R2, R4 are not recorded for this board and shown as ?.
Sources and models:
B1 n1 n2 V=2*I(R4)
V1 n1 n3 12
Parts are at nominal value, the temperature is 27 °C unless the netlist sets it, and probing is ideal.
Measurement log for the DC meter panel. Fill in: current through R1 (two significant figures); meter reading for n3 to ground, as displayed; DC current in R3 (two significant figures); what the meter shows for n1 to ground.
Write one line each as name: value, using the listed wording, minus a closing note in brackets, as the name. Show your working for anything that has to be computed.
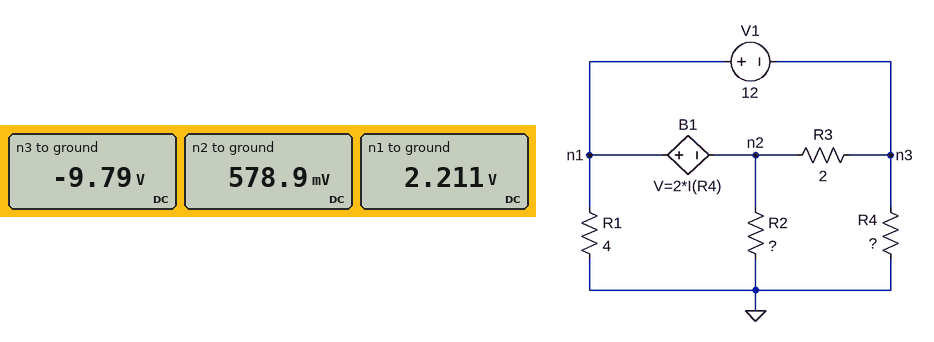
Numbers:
current through R1: (2.211 V) / 4 Ω = 550 mA
meter reading for n3 to ground, as displayed: -9.79 V
DC current in R3: (578.9 mV - (-9.79 V)) / 2 Ω = 5.2 A
what the meter shows for n1 to ground: 2.211 V
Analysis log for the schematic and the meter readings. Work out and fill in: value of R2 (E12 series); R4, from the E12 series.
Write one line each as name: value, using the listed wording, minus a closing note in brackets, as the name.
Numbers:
value of R2: 2.2 Ω
R4, from the E12 series: 12 Ω
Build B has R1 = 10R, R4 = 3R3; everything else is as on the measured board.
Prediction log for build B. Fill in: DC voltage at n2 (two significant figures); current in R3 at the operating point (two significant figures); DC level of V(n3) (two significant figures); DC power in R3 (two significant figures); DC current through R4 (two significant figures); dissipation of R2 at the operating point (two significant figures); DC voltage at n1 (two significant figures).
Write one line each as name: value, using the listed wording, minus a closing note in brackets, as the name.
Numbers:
DC voltage at n2: 2.6 V
current in R3 at the operating point: 4.2 A
DC level of V(n3): -5.9 V
DC power in R3: 36 W
DC current through R4: 1.8 A
dissipation of R2 at the operating point: 3.0 W
DC voltage at n1: 6.1 V
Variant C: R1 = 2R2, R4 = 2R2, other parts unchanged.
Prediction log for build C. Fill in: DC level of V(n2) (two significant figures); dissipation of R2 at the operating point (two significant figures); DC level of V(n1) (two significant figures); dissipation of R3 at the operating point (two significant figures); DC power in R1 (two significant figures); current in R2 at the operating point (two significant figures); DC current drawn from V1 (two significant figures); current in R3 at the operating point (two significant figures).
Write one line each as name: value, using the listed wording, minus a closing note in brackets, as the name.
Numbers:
DC level of V(n2): 280 mV
dissipation of R2 at the operating point: 35 mW
DC level of V(n1): 5.9 V
dissipation of R3 at the operating point: 21 W
DC power in R1: 16 W
current in R2 at the operating point: 130 mA
DC current drawn from V1: 6.0 A
current in R3 at the operating point: 3.2 A
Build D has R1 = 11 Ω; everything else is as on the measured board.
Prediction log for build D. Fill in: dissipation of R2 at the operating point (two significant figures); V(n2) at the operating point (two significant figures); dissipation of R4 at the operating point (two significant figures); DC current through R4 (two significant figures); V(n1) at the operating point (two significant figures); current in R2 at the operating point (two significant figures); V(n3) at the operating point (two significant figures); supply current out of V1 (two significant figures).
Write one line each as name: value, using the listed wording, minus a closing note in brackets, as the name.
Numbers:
dissipation of R2 at the operating point: 610 mW
V(n2) at the operating point: 1.2 V
dissipation of R4 at the operating point: 7.2 W
DC current through R4: 770 mA
V(n1) at the operating point: 2.7 V
current in R2 at the operating point: 530 mA
V(n3) at the operating point: -9.3 V
supply current out of V1: 6.0 A
